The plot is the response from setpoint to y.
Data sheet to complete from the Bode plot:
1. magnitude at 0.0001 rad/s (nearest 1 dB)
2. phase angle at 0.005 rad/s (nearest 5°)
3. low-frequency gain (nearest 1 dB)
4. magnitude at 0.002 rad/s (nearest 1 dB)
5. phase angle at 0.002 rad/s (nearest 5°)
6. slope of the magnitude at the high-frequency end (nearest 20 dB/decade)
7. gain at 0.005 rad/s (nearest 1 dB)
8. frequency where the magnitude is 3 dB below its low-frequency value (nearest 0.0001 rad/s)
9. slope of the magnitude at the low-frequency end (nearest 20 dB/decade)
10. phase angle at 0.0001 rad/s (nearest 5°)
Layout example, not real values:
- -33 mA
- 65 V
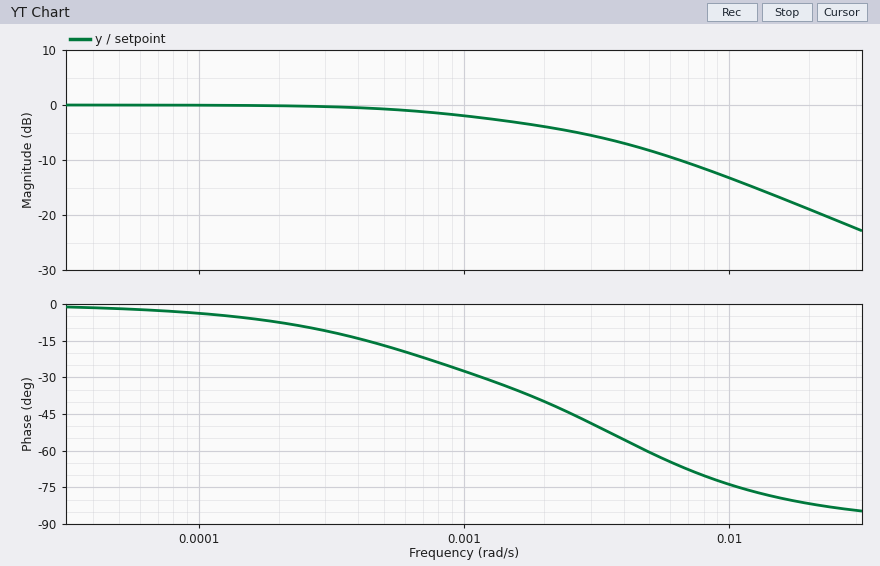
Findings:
- 0 dB
- -60°
- 0 dB
- -4 dB
- -40°
- -20 dB/decade
- -8 dB
- 0.0015 rad/s
- 0 dB/decade
- -5°
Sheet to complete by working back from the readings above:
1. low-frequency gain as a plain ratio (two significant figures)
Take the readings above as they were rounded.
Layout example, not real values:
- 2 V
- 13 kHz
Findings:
- 1.0
